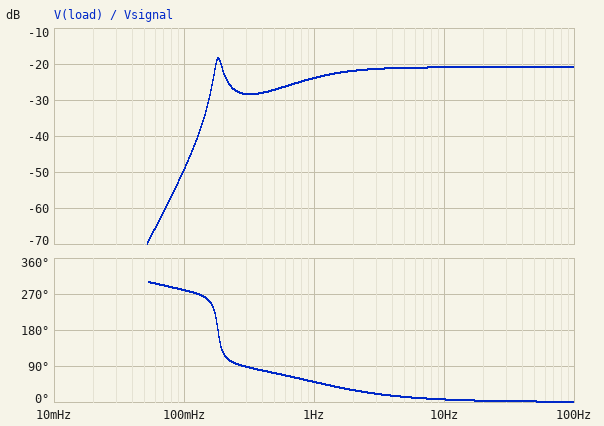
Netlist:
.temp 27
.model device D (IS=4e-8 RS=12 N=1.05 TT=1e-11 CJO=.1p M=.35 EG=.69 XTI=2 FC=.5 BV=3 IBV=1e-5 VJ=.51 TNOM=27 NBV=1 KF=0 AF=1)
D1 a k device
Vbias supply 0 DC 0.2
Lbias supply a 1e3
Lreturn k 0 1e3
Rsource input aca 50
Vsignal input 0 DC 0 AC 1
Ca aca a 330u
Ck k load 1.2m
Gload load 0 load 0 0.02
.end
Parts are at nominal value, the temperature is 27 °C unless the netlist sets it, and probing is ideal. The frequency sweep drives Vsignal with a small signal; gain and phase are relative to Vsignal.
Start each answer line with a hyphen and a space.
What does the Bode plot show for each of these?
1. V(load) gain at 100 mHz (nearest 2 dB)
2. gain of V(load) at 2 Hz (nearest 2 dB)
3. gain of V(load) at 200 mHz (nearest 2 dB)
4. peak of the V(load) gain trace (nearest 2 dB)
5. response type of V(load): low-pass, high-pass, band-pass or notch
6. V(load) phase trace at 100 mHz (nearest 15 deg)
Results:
- -50 dB
- -22 dB
- -22 dB
- -18 dB
- high-pass
- 285 deg
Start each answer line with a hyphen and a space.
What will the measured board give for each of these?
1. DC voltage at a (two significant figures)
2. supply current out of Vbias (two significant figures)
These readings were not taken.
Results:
- 200 mV
- 61 µA
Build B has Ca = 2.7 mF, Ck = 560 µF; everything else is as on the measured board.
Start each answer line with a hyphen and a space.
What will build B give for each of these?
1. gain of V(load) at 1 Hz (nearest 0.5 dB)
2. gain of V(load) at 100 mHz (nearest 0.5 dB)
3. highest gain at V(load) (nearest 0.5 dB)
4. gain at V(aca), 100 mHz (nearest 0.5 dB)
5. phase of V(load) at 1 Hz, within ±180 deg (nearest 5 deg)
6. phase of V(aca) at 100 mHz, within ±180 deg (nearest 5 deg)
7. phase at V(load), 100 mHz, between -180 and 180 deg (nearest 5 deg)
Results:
- -22.0 dB
- -32.5 dB
- -21.0 dB
- -1.0 dB
- 35 deg
- -10 deg
- -105 deg
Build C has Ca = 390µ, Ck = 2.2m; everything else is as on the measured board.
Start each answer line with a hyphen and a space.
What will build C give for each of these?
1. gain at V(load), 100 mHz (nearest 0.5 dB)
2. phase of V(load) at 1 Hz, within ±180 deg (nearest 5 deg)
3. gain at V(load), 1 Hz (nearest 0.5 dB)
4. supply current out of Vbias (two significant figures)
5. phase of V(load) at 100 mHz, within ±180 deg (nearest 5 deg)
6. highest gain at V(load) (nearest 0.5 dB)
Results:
- -39.5 dB
- 45 deg
- -23.0 dB
- 61 µA
- -95 deg
- -21.0 dB
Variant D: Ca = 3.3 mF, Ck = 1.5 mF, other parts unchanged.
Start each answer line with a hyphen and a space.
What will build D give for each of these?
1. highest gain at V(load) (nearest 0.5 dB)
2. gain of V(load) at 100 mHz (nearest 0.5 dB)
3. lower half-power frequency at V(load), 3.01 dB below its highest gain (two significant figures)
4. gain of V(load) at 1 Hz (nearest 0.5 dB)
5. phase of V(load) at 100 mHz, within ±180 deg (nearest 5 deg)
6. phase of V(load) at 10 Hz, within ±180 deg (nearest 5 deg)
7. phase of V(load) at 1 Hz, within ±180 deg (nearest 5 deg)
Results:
- -12.5 dB
- -13.5 dB
- 98 mHz
- -21.0 dB
- -155 deg
- 0 deg
- 15 deg
